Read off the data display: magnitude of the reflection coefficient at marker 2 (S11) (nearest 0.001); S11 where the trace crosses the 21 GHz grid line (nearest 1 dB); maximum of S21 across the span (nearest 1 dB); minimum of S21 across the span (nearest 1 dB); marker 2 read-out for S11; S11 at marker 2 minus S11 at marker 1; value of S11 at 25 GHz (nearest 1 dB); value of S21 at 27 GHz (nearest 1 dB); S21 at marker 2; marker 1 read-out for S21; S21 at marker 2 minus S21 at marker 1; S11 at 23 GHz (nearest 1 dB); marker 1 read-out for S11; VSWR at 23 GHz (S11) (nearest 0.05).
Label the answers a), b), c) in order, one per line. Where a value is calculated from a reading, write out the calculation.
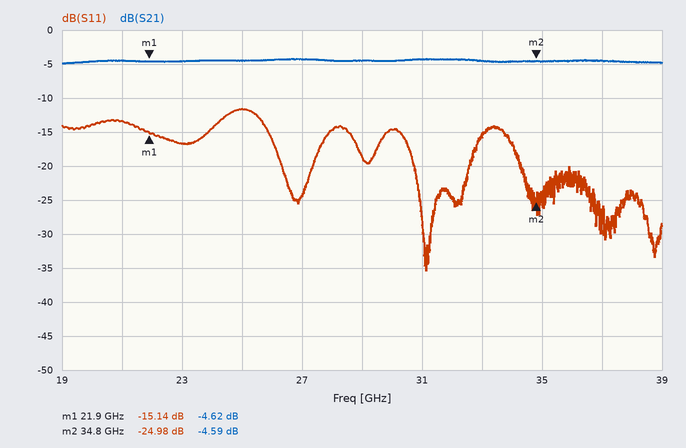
a) 10^(-24.98/20) ≈ 0.056
b) -13 dB
c) -4 dB
d) -5 dB
e) -24.98 dB
f) -24.98 − (-15.14) = -9.84 dB
g) -12 dB
h) -4 dB
i) -4.59 dB
j) -4.62 dB
k) -4.59 − (-4.62) = 0.03 dB
l) -17 dB
m) -15.14 dB
n) |Γ| = 10^(-17/20) = 0.1413; VSWR = (1 + 0.1413)/(1 − 0.1413) ≈ 1.33, so 1.35 to the nearest 0.05
